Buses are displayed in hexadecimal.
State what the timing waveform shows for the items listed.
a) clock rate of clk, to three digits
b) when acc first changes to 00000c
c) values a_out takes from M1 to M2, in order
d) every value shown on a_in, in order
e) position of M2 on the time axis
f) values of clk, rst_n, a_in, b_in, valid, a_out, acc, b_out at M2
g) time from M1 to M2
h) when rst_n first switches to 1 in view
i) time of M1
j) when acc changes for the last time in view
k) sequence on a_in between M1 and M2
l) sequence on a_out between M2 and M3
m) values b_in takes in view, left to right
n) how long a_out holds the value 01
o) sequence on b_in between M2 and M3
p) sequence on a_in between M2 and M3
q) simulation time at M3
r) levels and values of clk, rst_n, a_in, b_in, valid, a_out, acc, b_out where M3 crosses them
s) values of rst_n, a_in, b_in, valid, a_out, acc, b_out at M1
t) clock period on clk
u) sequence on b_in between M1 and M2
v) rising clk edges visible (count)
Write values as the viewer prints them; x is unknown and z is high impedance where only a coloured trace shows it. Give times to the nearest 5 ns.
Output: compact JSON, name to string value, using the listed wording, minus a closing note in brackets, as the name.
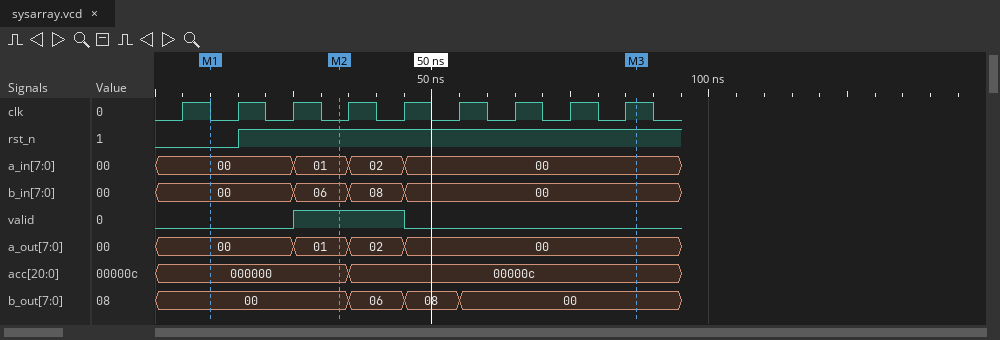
{"clock rate of clk, to three digits": "100 MHz", "when acc first changes to 00000c": "35 ns", "values a_out takes from M1 to M2, in order": "00, 01", "every value shown on a_in, in order": "00, 01, 02, 00", "position of M2 on the time axis": "35 ns", "values of clk, rst_n, a_in, b_in, valid, a_out, acc, b_out at M2": "clk=0, rst_n=1, a_in=01, b_in=06, valid=1, a_out=01, acc=000000, b_out=00", "time from M1 to M2": "25 ns", "when rst_n first switches to 1 in view": "15 ns", "time of M1": "10 ns", "when acc changes for the last time in view": "35 ns", "sequence on a_in between M1 and M2": "00, 01", "sequence on a_out between M2 and M3": "01, 02, 00", "values b_in takes in view, left to right": "00, 06, 08, 00", "how long a_out holds the value 01": "10 ns", "sequence on b_in between M2 and M3": "06, 08, 00", "sequence on a_in between M2 and M3": "01, 02, 00", "simulation time at M3": "85 ns", "levels and values of clk, rst_n, a_in, b_in, valid, a_out, acc, b_out where M3 crosses them": "clk=1, rst_n=1, a_in=00, b_in=00, valid=0, a_out=00, acc=00000c, b_out=00", "values of rst_n, a_in, b_in, valid, a_out, acc, b_out at M1": "rst_n=0, a_in=00, b_in=00, valid=0, a_out=00, acc=000000, b_out=00", "clock period on clk": "10 ns", "sequence on b_in between M1 and M2": "00, 06", "rising clk edges visible": "9"}
